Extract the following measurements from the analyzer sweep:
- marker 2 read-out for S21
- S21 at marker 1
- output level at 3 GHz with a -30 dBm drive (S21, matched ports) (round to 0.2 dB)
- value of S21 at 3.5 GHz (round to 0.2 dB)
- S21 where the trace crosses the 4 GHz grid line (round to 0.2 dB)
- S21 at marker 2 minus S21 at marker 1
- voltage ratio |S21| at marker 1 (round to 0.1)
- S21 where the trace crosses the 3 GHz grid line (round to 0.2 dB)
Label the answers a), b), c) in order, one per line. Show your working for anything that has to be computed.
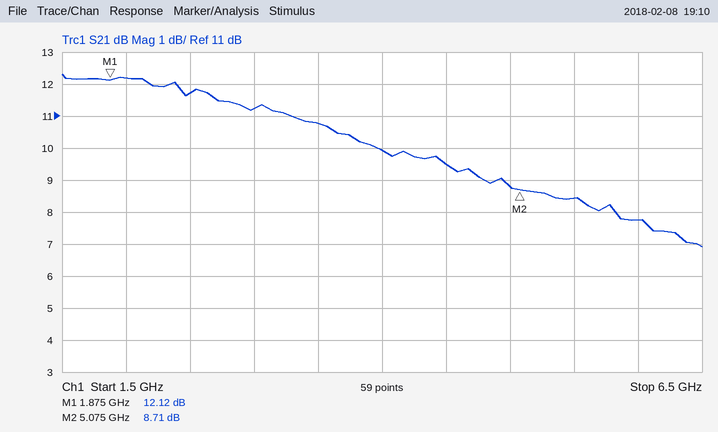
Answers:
a) 8.71 dB
b) 12.12 dB
c) -30 dBm + (11.2 dB) = -18.8 dBm
d) 10.8 dB
e) 10.0 dB
f) 8.71 − (12.12) = -3.41 dB
g) 10^(12.12/20) ≈ 4.0
h) 11.2 dB
